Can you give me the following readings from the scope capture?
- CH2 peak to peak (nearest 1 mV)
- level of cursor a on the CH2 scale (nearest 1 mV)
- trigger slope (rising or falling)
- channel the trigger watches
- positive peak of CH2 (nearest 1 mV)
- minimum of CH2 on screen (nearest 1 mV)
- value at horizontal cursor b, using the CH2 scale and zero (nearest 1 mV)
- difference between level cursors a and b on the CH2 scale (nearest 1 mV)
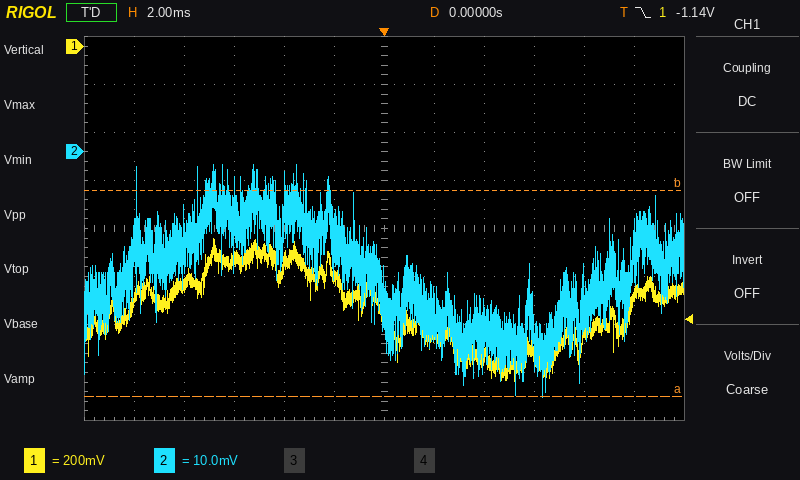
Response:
48 mV
-51 mV
falling
CH1
-3 mV
-51 mV
-8 mV
43 mV
